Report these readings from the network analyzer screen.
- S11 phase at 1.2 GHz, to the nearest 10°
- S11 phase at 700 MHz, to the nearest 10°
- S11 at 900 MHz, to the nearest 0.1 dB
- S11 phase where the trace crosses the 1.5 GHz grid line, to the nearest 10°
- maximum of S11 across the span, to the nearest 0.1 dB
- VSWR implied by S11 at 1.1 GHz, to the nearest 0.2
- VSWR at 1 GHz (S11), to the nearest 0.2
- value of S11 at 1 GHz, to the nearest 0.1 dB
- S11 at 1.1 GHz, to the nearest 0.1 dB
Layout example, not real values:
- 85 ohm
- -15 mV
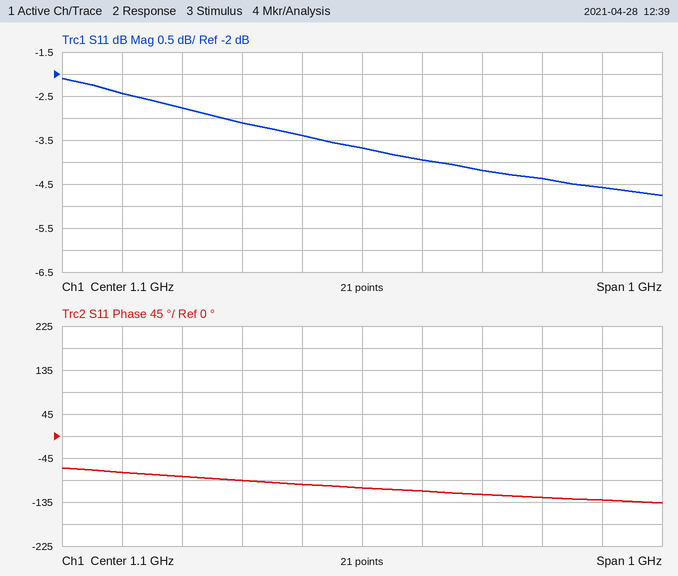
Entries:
- -110°
- -70°
- -3.1 dB
- -130°
- -2.1 dB
- 4.8
- 5.2
- -3.4 dB
- -3.7 dB
